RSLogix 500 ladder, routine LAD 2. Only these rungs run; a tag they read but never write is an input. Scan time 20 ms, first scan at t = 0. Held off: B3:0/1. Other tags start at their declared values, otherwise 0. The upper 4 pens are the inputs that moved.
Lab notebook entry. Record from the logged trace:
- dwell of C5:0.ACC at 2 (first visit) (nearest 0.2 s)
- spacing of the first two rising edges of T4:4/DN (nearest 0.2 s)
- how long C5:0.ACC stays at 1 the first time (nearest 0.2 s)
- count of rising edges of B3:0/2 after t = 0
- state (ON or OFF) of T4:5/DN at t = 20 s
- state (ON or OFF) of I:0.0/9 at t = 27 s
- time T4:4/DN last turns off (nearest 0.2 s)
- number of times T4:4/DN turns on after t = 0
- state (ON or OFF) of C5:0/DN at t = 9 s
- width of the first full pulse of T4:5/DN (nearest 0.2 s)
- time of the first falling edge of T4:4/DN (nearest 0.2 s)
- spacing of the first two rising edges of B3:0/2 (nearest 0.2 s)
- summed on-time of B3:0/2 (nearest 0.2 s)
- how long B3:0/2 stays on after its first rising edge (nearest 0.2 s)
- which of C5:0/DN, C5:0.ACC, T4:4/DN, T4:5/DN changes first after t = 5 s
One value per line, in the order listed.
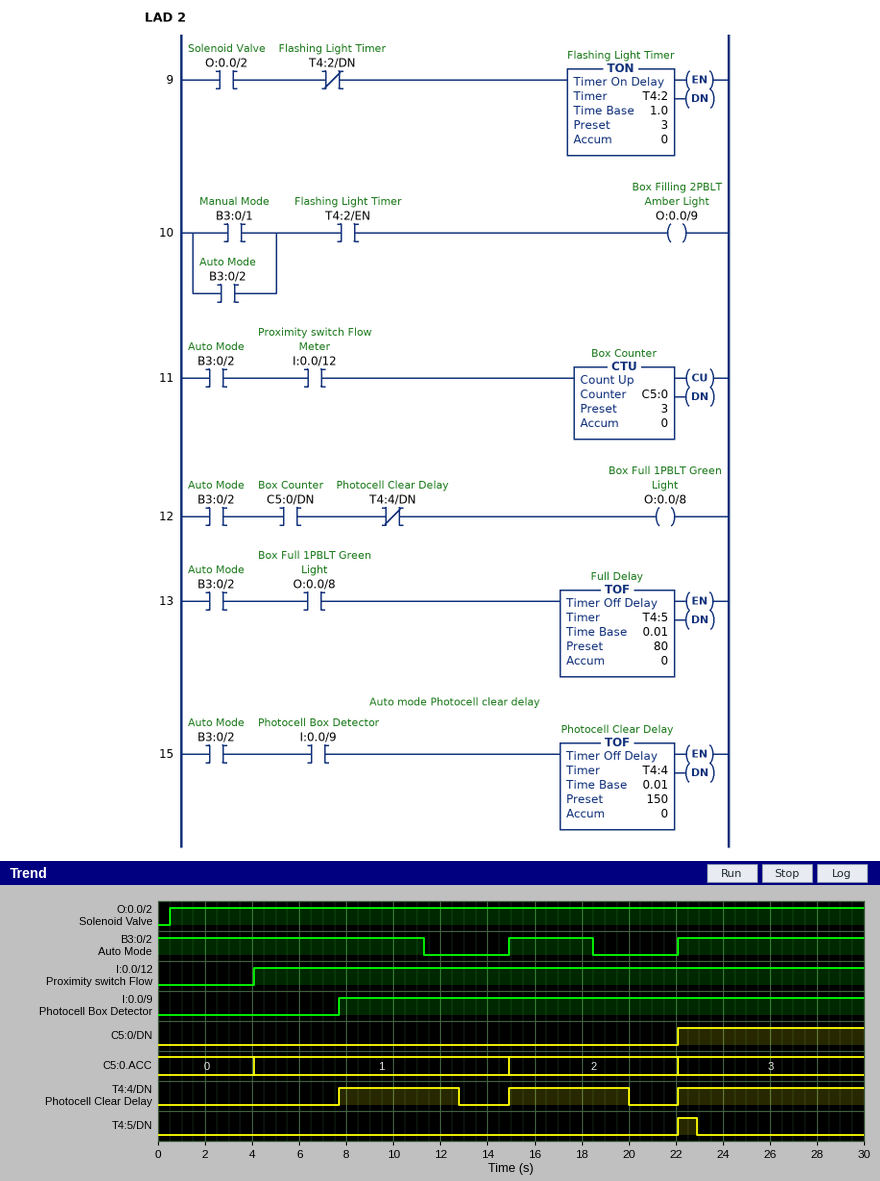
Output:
7.2 s
7.2 s
10.8 s
2
OFF
ON
20.0 s
3
OFF
0.8 s
12.8 s
7.2 s
22.8 s
3.6 s
T4:4/DN
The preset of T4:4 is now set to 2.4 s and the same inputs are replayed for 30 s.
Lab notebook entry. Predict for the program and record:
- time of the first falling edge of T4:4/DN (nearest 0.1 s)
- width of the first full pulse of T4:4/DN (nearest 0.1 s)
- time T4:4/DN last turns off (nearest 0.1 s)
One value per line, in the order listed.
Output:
13.7 s
6.0 s
20.9 s
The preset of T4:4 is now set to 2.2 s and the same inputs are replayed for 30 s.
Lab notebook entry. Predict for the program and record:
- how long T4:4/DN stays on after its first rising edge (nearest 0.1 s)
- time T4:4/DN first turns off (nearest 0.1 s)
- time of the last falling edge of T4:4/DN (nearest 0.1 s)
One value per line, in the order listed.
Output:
5.8 s
13.5 s
20.7 s
